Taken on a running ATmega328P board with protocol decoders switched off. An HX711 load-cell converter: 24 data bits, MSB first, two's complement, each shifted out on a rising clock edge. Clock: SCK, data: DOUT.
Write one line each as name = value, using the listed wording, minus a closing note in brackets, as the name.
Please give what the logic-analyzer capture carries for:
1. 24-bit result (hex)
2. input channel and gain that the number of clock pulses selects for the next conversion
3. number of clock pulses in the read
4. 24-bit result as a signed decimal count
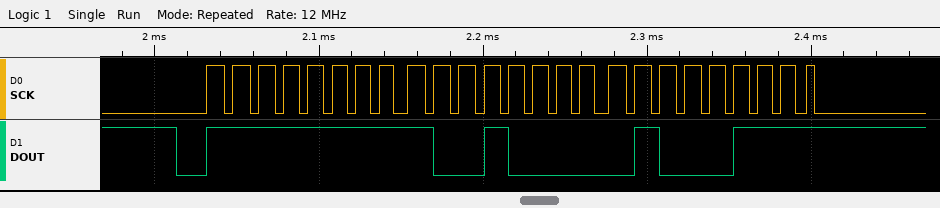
24-bit result = 0xFF9047
input channel and gain that the number of clock pulses selects for the next conversion = channel A, gain 128
number of clock pulses in the read = 25
24-bit result as a signed decimal count = -28601
